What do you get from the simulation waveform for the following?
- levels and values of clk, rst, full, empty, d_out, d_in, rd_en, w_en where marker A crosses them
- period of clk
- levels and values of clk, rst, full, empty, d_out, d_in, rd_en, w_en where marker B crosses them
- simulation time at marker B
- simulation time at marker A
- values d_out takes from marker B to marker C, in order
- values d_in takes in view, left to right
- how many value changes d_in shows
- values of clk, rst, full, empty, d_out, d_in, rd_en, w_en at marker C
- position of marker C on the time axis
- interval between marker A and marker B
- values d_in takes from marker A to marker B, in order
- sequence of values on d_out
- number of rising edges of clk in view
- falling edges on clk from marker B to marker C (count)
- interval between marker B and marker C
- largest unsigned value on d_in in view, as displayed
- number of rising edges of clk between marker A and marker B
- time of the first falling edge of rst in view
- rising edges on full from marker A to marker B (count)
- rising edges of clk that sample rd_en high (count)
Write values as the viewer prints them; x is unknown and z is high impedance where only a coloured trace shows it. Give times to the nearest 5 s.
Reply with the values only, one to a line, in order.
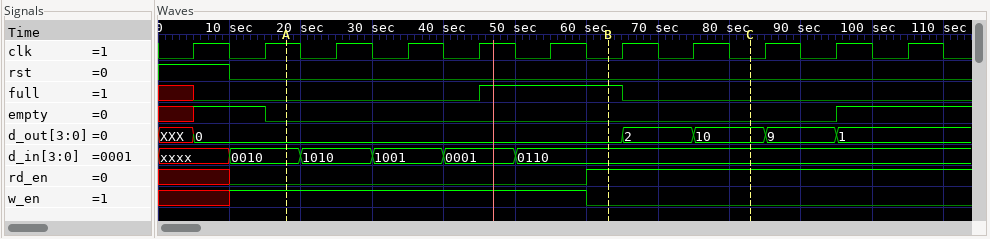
clk=1, rst=0, full=0, empty=0, d_out=0, d_in=0010, rd_en=0, w_en=1
10 s
clk=0, rst=0, full=1, empty=0, d_out=0, d_in=0110, rd_en=1, w_en=0
65 s
20 s
0, 2, 10
xxxx, 0010, 1010, 1001, 0001, 0110
5
clk=0, rst=0, full=0, empty=0, d_out=10, d_in=0110, rd_en=1, w_en=0
85 s
45 s
0010, 1010, 1001, 0001, 0110
XXX, 0, 2, 10, 9, 1
11
2
20 s
1010
4
10 s
1
5
